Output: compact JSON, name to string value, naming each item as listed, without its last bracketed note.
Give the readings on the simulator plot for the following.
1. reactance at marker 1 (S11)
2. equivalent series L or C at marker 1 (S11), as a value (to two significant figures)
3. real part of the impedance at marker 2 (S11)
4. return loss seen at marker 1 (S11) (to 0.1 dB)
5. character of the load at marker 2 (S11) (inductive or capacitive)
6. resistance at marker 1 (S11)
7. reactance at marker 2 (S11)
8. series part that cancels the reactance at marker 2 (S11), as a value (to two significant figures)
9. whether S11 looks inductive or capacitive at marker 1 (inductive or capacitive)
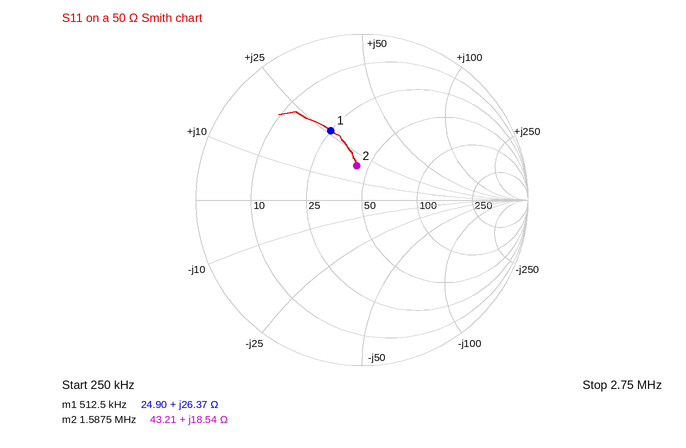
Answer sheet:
{"reactance at marker 1": "+26.37 Ω", "equivalent series L or C at marker 1 (S11), as a value": "8.2 µH", "real part of the impedance at marker 2": "43.21 Ω", "return loss seen at marker 1 (S11)": "6.8 dB", "character of the load at marker 2 (S11)": "inductive", "resistance at marker 1": "24.90 Ω", "reactance at marker 2": "+18.54 Ω", "series part that cancels the reactance at marker 2 (S11), as a value": "5.4 nF", "whether S11 looks inductive or capacitive at marker 1": "inductive"}
